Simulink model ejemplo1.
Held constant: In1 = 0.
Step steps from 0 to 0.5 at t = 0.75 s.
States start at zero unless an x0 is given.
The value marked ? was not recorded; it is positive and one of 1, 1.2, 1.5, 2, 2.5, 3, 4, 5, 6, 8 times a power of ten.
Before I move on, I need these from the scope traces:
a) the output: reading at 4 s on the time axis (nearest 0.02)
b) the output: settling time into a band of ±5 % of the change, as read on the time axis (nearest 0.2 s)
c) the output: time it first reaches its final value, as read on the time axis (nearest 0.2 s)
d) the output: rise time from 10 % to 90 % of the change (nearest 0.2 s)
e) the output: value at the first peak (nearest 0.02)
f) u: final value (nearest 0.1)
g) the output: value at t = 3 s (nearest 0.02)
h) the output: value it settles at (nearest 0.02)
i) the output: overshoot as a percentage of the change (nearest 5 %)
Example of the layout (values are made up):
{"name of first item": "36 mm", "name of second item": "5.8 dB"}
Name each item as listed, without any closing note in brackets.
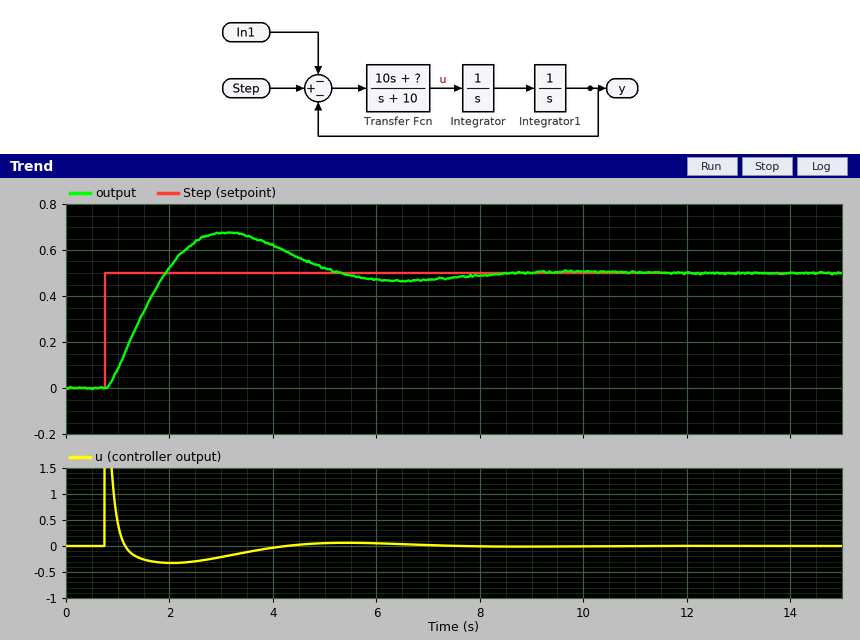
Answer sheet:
{"the output: reading at 4 s on the time axis": "0.62", "the output: settling time into a band of ±5 % of the change, as read on the time axis": "7.2 s", "the output: time it first reaches its final value, as read on the time axis": "2.0 s", "the output: rise time from 10 % to 90 % of the change": "0.8 s", "the output: value at the first peak": "0.68", "u: final value": "0.0", "the output: value at t = 3 s": "0.68", "the output: value it settles at": "0.50", "the output: overshoot as a percentage of the change": "35 %"}
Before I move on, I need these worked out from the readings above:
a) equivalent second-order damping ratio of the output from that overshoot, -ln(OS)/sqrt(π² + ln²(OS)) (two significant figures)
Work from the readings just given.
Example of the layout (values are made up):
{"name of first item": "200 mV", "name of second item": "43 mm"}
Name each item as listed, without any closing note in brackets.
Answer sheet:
{"equivalent second-order damping ratio of the output from that overshoot, -ln(OS)/sqrt(π² + ln²(OS))": "0.32"}
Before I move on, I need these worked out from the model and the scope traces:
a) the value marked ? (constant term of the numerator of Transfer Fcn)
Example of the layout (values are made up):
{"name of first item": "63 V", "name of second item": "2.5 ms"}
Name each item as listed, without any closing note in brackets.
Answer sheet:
{"the value marked ?": "10"}
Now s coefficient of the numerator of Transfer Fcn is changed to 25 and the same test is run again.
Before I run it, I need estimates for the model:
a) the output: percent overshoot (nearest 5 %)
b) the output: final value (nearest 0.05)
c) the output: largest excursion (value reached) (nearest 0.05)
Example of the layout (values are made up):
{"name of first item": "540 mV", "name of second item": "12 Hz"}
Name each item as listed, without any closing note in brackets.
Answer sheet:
{"the output: percent overshoot": "10 %", "the output: final value": "0.50", "the output: largest excursion (value reached)": "0.55"}
